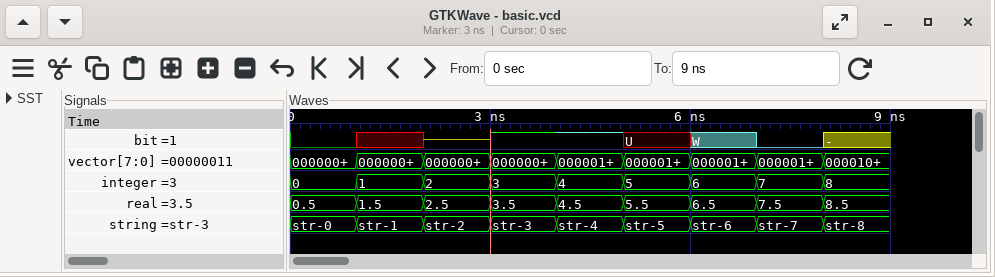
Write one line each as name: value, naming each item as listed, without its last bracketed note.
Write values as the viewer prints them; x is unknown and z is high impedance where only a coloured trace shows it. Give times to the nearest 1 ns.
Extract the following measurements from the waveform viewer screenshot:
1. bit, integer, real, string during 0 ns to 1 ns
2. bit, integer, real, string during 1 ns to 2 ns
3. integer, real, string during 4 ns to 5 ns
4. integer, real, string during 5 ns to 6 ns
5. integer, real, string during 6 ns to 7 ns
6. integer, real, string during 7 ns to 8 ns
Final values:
bit, integer, real, string during 0 ns to 1 ns: bit=0, integer=0, real=0.5, string=str-0
bit, integer, real, string during 1 ns to 2 ns: bit=x, integer=1, real=1.5, string=str-1
integer, real, string during 4 ns to 5 ns: integer=4, real=4.5, string=str-4
integer, real, string during 5 ns to 6 ns: integer=5, real=5.5, string=str-5
integer, real, string during 6 ns to 7 ns: integer=6, real=6.5, string=str-6
integer, real, string during 7 ns to 8 ns: integer=7, real=7.5, string=str-7
